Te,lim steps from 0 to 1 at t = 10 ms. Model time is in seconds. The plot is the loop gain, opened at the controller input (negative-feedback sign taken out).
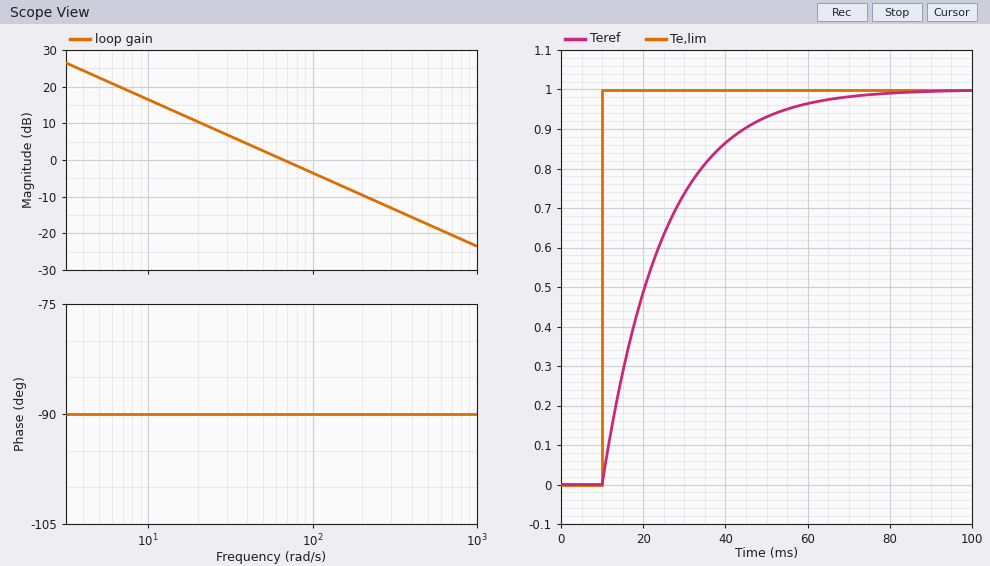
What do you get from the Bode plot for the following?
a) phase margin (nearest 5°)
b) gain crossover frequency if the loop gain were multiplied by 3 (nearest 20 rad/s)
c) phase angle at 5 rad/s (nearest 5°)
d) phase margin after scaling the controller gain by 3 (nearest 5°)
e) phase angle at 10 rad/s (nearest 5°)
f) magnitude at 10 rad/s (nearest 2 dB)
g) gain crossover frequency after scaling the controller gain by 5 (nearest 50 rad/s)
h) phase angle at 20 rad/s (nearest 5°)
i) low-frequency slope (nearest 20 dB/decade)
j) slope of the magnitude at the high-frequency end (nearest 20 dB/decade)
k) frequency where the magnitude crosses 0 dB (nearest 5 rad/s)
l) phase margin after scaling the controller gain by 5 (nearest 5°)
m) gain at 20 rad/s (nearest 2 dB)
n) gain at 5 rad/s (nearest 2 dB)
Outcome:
90°
200 rad/s
-90°
90°
-90°
16 dB
350 rad/s
-90°
-20 dB/decade
-20 dB/decade
65 rad/s
90°
10 dB
22 dB
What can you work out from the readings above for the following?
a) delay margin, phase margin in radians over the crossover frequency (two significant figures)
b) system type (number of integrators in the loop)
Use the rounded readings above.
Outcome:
0.024 s
1
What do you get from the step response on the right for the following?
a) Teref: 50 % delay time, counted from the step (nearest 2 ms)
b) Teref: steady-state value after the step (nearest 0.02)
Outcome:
10 ms
1.00
